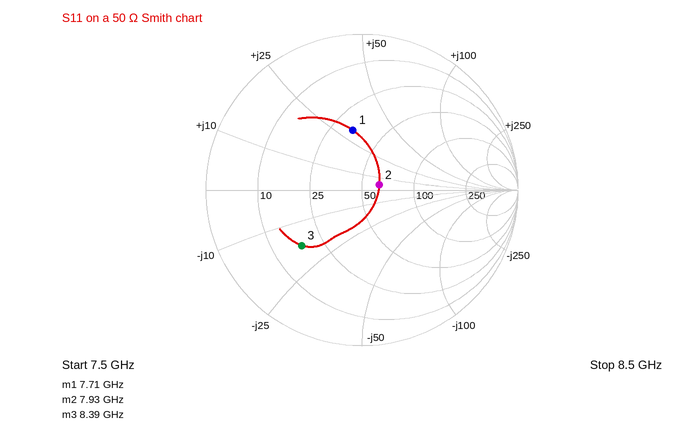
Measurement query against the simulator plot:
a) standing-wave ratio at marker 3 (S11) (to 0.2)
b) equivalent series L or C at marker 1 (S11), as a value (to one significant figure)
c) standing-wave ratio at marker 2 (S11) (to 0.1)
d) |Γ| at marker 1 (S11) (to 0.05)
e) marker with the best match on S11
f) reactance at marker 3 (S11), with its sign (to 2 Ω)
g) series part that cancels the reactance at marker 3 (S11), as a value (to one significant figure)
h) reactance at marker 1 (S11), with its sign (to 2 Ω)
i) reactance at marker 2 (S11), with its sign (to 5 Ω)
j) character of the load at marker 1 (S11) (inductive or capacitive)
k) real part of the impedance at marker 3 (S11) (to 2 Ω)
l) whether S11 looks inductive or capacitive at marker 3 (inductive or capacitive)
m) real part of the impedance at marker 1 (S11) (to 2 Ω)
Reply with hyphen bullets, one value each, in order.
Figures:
- 3.2
- 600 pH
- 1.3
- 0.40
- marker 2
- -18 Ω
- 300 pH
- +30 Ω
- +5 Ω
- inductive
- 18 Ω
- capacitive
- 34 Ω
